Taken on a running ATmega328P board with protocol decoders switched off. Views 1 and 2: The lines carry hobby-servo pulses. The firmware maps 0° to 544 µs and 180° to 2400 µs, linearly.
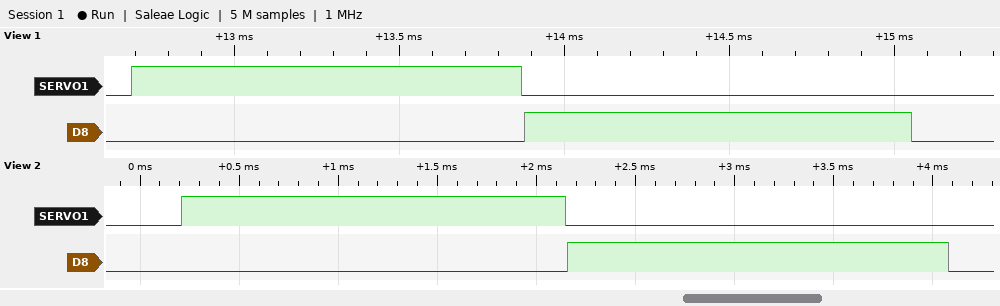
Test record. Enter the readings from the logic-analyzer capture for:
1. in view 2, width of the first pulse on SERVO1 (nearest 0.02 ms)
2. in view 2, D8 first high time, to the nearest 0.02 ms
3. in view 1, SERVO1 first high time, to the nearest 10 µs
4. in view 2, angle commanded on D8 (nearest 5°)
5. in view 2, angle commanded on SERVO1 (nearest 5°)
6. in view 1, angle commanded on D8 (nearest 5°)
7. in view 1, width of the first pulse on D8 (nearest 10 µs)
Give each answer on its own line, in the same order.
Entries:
1.94 ms
1.92 ms
1180 µs
135°
135°
60°
1170 µs
